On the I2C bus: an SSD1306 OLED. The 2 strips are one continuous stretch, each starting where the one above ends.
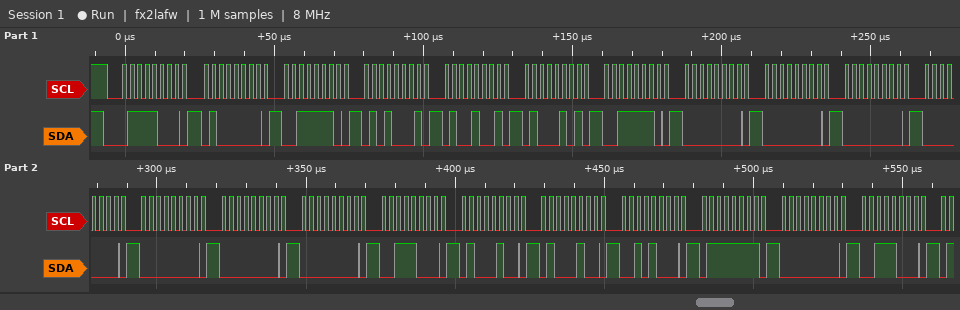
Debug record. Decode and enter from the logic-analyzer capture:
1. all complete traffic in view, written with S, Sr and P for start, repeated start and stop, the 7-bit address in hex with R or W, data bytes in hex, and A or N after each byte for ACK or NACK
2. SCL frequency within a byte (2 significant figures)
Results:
S 3CW A 40 A 3E A 51 A 49 A 45 A 3E A 00 A 00 A 00 A 00 A 00 A 00 A 00 A 38 A 44 A 44 A 28 A 7F A 00 A 38 A
400 kHz
